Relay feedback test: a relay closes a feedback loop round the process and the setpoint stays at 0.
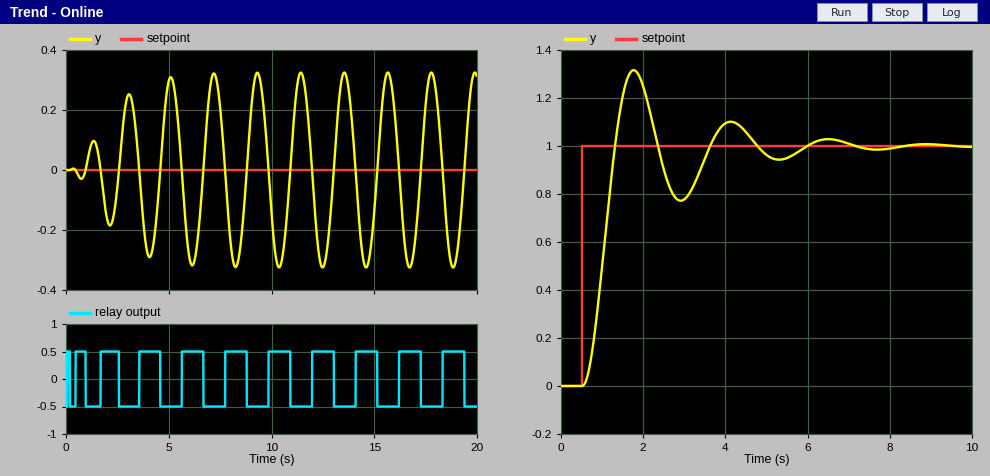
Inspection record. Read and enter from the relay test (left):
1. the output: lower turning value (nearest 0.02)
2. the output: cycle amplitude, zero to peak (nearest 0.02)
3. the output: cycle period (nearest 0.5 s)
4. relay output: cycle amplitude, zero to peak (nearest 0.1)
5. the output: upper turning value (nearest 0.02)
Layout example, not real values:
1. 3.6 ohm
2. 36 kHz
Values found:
1. -0.32
2. 0.32
3. 2.0 s
4. 0.5
5. 0.32
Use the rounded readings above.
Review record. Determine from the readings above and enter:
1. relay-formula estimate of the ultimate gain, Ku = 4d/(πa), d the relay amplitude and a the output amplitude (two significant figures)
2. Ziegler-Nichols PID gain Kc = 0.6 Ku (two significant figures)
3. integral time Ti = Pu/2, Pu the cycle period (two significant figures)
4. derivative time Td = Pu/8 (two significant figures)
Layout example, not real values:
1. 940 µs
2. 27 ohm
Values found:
1. 2.0
2. 1.2
3. 1.0 s
4. 0.25 s
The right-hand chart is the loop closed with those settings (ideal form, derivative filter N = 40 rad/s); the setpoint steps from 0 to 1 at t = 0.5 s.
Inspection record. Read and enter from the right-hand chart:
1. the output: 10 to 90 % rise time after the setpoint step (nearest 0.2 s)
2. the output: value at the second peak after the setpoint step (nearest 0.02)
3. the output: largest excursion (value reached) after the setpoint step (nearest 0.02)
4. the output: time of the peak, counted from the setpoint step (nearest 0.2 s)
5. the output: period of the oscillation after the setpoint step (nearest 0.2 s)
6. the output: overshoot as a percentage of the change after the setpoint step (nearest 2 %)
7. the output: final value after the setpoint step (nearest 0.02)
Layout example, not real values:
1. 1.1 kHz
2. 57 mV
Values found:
1. 0.6 s
2. 1.10
3. 1.32
4. 1.2 s
5. 2.4 s
6. 32 %
7. 1.00
